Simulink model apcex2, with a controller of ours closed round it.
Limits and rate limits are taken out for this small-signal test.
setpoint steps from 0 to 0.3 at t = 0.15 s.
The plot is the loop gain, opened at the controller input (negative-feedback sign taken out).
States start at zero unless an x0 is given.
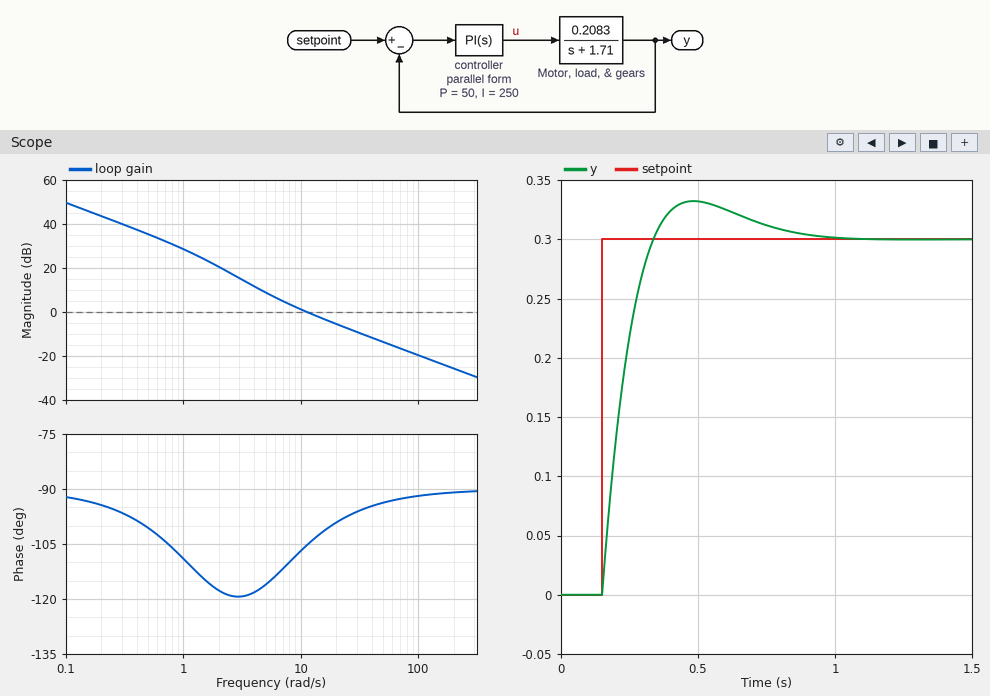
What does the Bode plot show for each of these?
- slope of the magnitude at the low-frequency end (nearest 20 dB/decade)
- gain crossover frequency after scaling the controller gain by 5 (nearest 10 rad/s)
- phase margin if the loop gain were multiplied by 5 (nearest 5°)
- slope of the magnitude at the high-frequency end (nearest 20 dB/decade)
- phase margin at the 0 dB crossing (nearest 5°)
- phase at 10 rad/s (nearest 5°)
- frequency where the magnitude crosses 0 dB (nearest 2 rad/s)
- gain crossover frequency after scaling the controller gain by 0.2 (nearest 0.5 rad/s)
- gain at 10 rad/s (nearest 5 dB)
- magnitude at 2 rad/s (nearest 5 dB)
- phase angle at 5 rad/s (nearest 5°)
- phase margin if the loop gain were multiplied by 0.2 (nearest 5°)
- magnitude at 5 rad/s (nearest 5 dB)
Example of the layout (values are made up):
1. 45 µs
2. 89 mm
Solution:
1. -20 dB/decade
2. 50 rad/s
3. 85°
4. -20 dB/decade
5. 75°
6. -105°
7. 12 rad/s
8. 3.5 rad/s
9. 0 dB
10. 20 dB
11. -115°
12. 60°
13. 10 dB
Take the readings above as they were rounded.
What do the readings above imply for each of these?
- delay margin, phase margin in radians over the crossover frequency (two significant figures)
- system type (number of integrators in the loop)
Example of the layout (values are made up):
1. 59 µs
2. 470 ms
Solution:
1. 0.11 s
2. 1
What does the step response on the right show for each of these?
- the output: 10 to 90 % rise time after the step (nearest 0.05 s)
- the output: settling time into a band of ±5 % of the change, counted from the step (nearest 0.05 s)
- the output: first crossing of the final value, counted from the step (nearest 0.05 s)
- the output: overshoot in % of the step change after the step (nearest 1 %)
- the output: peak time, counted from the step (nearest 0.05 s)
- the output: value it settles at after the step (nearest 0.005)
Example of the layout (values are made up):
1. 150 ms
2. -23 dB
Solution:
1. 0.15 s
2. 0.55 s
3. 0.20 s
4. 11 %
5. 0.35 s
6. 0.300
